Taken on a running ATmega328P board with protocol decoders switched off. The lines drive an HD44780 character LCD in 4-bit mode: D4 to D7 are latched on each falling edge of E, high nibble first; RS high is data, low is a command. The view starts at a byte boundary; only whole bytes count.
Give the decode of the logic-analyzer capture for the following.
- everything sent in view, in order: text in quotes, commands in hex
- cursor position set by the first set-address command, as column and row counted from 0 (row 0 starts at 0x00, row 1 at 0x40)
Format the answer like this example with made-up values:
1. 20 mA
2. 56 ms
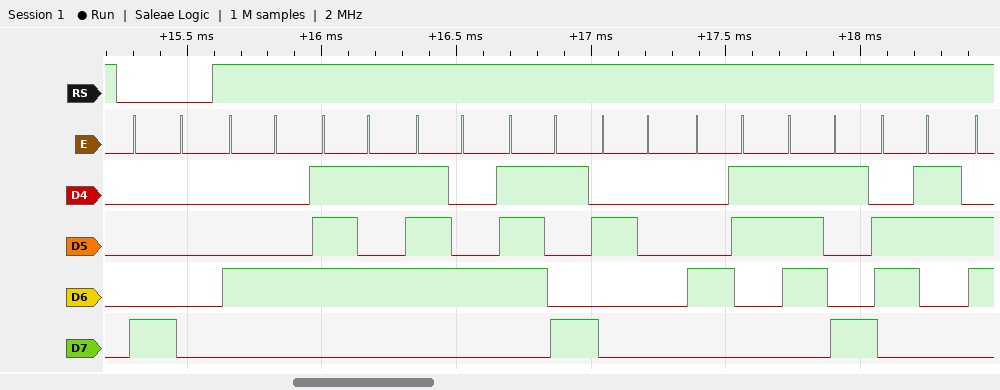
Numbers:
1. 0x80 "Duty Cyc"
2. column 0, row 0
